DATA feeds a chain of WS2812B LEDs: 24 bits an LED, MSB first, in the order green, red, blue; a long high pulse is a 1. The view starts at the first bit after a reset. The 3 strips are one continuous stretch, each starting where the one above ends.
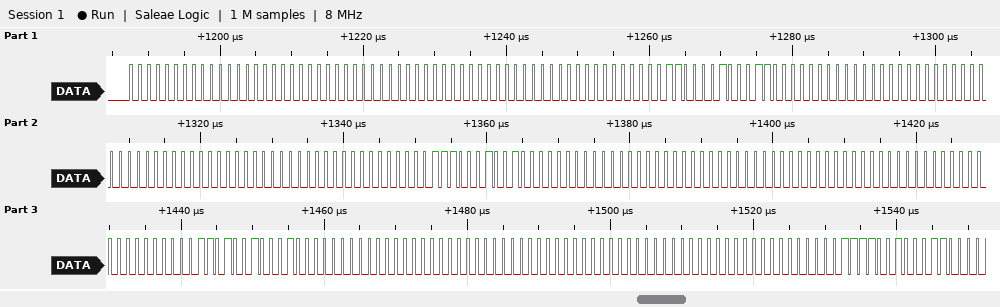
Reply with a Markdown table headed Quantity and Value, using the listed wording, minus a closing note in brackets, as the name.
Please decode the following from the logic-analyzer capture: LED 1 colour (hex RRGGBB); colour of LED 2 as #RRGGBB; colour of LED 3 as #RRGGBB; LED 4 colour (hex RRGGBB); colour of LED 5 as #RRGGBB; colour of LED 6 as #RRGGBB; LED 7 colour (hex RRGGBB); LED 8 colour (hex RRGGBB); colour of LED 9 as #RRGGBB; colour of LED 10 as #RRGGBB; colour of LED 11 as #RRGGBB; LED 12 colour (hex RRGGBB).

| Quantity | Value |
|---|---|
| LED 1 colour | #000000 |
| colour of LED 2 as #RRGGBB | #000000 |
| colour of LED 3 as #RRGGBB | #0C0023 |
| LED 4 colour | #000000 |
| colour of LED 5 as #RRGGBB | #000000 |
| colour of LED 6 as #RRGGBB | #0E0024 |
| LED 7 colour | #000000 |
| LED 8 colour | #000000 |
| colour of LED 9 as #RRGGBB | #0D0022 |
| colour of LED 10 as #RRGGBB | #000000 |
| colour of LED 11 as #RRGGBB | #000000 |
| LED 12 colour | #0F0023 |
